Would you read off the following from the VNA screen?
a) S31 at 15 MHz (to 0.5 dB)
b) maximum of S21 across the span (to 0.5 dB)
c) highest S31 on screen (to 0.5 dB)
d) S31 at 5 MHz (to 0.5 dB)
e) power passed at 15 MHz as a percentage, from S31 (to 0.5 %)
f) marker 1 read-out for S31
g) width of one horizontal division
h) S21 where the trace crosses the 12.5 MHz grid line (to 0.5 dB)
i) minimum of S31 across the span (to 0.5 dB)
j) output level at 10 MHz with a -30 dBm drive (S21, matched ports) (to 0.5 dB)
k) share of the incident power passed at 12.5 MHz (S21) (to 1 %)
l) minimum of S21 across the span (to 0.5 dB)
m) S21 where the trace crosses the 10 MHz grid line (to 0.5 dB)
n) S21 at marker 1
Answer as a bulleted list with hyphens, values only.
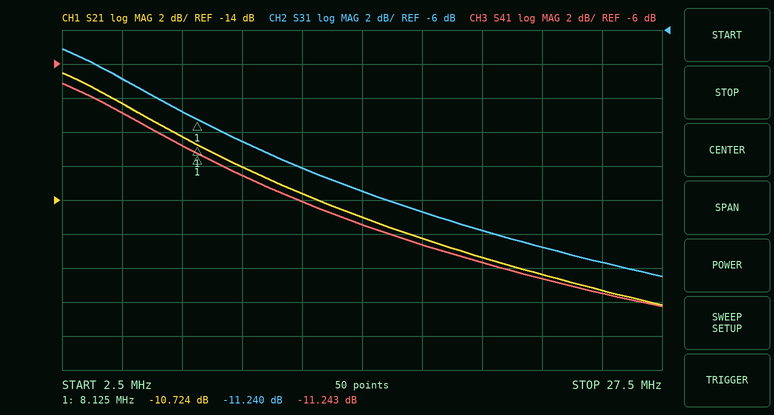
- -15.5 dB
- -6.5 dB
- -7.0 dB
- -9.0 dB
- 3.0 %
- -11.240 dB
- 2.5 MHz
- -13.5 dB
- -20.5 dB
- -42.0 dBm
- 4 %
- -20.0 dB
- -12.0 dB
- -10.724 dB
